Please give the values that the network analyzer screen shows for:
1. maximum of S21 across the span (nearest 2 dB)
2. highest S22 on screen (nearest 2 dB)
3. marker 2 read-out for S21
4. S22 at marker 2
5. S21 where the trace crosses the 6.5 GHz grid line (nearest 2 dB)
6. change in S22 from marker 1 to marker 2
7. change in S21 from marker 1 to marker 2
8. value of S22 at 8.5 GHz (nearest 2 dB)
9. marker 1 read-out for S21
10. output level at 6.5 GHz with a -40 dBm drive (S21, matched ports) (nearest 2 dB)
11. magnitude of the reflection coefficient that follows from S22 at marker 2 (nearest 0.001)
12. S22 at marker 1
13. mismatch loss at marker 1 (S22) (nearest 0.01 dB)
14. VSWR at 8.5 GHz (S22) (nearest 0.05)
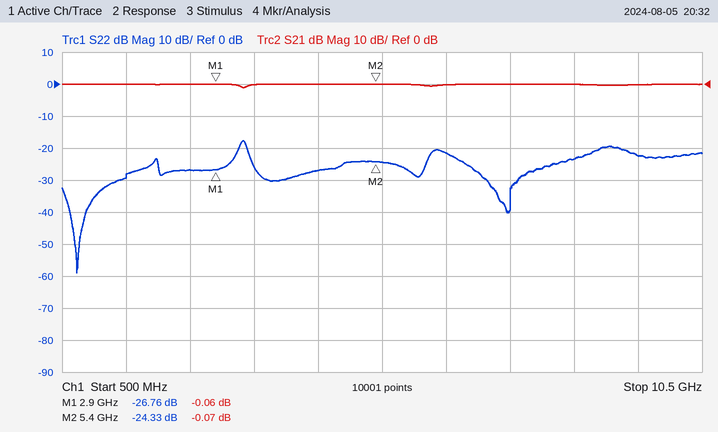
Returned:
0 dB
-18 dB
-0.07 dB
-24.33 dB
0 dB
2.43 dB
-0.01 dB
-24 dB
-0.06 dB
-40 dBm
0.061
-26.76 dB
0.01 dB
1.15
